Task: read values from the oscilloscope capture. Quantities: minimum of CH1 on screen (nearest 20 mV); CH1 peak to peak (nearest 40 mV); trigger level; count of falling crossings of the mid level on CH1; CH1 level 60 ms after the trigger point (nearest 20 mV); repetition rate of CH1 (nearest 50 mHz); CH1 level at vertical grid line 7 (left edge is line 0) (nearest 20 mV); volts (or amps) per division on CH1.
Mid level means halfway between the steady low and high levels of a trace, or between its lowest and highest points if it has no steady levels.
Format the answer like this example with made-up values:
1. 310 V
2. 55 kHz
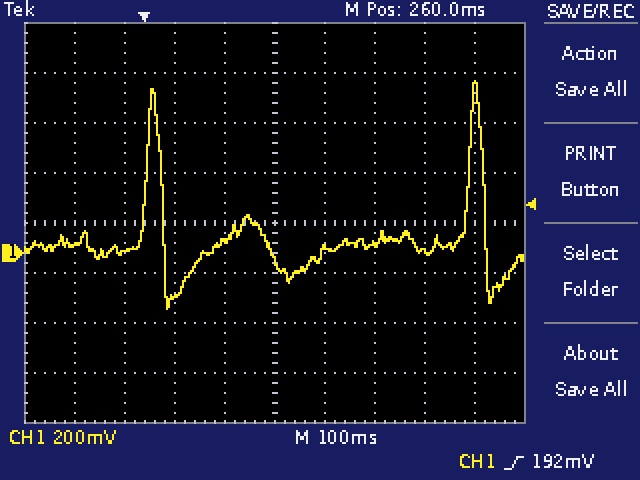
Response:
1. -220 mV
2. 920 mV
3. 192 mV
4. 2
5. -180 mV
6. 1.55 Hz
7. 40 mV
8. 200 mV
